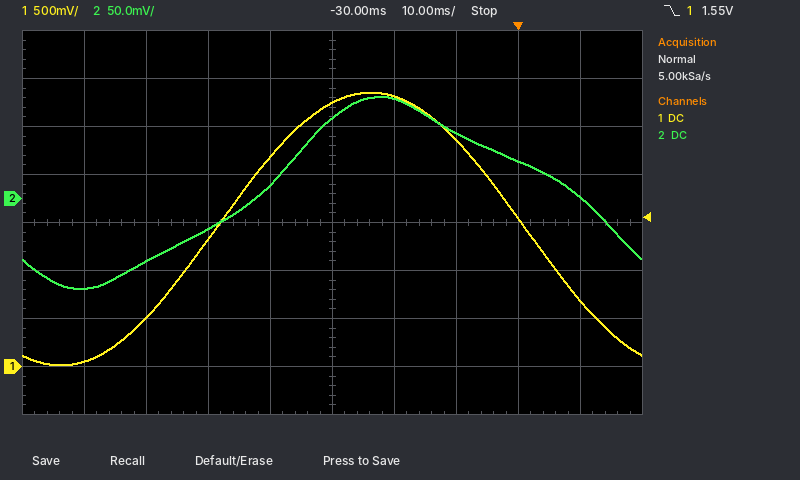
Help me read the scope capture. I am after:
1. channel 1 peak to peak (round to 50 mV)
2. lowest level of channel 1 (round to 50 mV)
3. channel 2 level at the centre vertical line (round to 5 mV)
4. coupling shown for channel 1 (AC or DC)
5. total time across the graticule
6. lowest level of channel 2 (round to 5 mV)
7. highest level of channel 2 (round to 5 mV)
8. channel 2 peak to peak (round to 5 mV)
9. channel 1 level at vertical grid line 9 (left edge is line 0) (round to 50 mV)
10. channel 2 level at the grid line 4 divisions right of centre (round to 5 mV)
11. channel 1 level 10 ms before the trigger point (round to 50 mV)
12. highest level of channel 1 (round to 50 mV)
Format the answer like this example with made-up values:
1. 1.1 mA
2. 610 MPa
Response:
1. 2.85 V
2. 0 mV
3. 85 mV
4. DC
5. 100 ms
6. -95 mV
7. 105 mV
8. 200 mV
9. 700 mV
10. 0 mV
11. 2.35 V
12. 2.85 V
